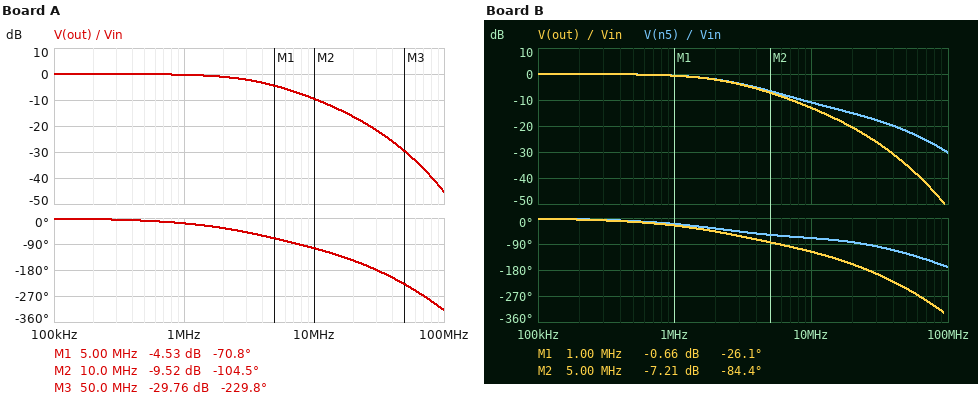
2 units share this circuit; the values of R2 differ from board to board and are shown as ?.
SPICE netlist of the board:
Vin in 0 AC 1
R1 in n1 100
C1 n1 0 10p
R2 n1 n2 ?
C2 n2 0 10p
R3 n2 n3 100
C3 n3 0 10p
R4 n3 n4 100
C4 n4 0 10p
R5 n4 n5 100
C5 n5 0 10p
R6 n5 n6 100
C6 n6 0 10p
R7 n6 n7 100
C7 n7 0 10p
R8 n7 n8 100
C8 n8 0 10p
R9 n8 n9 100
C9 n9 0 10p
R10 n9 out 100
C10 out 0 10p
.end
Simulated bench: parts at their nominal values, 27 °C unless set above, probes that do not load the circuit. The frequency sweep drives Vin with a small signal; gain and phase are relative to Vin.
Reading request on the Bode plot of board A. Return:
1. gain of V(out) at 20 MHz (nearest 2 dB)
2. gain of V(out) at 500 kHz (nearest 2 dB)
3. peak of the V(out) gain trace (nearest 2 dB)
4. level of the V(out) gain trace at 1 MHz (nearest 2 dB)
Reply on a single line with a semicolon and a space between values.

-16 dB; 0 dB; 0 dB; 0 dB
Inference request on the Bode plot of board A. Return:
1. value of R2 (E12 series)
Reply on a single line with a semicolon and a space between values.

68 Ω
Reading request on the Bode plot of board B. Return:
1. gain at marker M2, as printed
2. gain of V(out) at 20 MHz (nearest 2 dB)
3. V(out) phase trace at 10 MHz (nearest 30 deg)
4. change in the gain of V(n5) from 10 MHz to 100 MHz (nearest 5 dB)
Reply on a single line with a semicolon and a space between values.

-7.21 dB; -20 dB; -120 deg; -20 dB
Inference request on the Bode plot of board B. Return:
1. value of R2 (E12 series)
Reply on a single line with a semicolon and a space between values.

330 Ω
